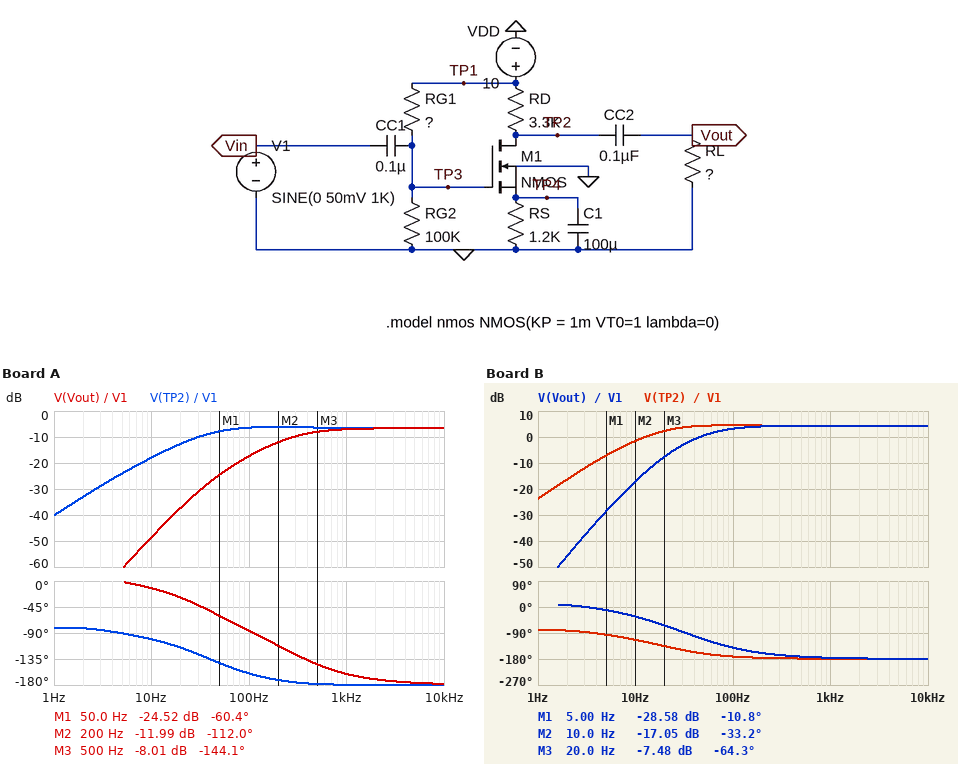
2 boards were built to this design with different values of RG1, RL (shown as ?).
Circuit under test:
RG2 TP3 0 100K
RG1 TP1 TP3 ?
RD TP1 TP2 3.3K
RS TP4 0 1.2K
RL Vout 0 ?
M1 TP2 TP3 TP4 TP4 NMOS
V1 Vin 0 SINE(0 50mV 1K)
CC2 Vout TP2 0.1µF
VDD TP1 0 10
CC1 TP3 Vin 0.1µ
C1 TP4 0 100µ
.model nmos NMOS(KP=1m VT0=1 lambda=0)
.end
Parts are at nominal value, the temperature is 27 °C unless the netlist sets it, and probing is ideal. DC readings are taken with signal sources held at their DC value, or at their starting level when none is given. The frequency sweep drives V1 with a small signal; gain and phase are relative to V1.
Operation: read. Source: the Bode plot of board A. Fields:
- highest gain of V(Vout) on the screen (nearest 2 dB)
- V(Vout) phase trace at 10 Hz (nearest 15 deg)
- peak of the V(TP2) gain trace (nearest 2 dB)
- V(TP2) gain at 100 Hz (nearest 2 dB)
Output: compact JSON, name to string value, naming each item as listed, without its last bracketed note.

{"highest gain of V(Vout) on the screen": "-6 dB", "V(Vout) phase trace at 10 Hz": "-15 deg", "peak of the V(TP2) gain trace": "-6 dB", "V(TP2) gain at 100 Hz": "-6 dB"}
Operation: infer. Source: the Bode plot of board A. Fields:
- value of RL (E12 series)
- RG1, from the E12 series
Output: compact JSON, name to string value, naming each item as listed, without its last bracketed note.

{"value of RL": "4.7 kΩ", "RG1, from the E12 series": "68 kΩ"}
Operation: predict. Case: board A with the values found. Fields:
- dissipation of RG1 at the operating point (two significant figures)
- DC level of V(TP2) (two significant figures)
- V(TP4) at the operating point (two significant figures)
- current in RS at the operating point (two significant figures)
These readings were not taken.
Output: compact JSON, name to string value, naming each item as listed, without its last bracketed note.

{"dissipation of RG1 at the operating point": "240 µW", "DC level of V(TP2)": "3.4 V", "V(TP4) at the operating point": "2.4 V", "current in RS at the operating point": "2.0 mA"}
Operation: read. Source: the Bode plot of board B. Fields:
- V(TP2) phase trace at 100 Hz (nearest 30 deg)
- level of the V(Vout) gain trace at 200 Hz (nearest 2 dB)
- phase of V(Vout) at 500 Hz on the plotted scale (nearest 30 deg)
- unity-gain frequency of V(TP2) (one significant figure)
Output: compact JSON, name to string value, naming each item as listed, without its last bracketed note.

{"V(TP2) phase trace at 100 Hz": "-180 deg", "level of the V(Vout) gain trace at 200 Hz": "4 dB", "phase of V(Vout) at 500 Hz on the plotted scale": "-180 deg", "unity-gain frequency of V(TP2)": "10 Hz"}
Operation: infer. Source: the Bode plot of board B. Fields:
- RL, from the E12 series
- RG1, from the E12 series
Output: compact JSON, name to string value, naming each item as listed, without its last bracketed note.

{"RL, from the E12 series": "27 kΩ", "RG1, from the E12 series": "470 kΩ"}
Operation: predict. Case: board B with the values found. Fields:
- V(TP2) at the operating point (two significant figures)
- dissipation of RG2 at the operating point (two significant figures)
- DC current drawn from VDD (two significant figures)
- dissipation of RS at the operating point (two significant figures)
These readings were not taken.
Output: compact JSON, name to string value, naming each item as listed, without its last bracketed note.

{"V(TP2) at the operating point": "9.5 V", "dissipation of RG2 at the operating point": "31 µW", "DC current drawn from VDD": "180 µA", "dissipation of RS at the operating point": "30 µW"}
